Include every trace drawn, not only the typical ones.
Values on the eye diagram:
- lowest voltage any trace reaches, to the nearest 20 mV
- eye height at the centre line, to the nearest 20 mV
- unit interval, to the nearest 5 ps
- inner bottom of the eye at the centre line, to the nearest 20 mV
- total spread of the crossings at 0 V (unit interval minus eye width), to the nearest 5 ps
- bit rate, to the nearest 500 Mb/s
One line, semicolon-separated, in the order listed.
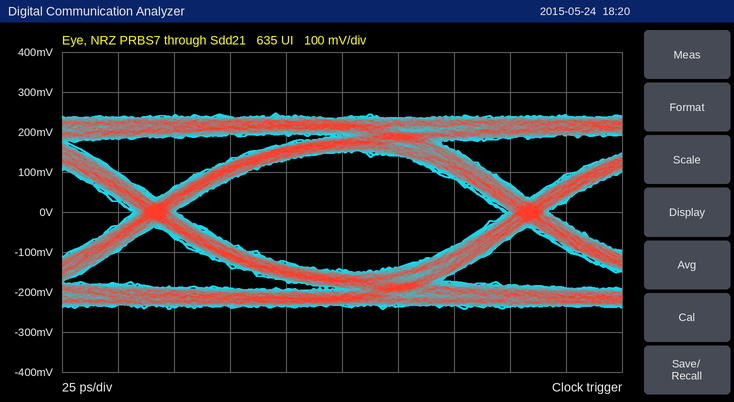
-240 mV; 300 mV; 165 ps; -140 mV; 20 ps; 6.0 Gb/s
